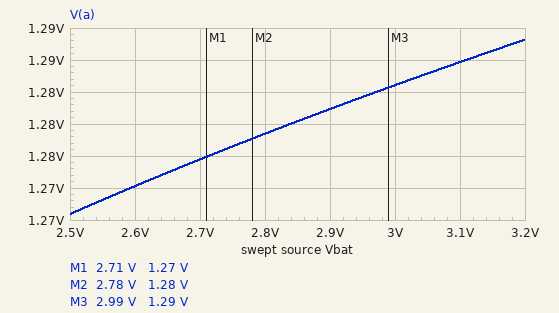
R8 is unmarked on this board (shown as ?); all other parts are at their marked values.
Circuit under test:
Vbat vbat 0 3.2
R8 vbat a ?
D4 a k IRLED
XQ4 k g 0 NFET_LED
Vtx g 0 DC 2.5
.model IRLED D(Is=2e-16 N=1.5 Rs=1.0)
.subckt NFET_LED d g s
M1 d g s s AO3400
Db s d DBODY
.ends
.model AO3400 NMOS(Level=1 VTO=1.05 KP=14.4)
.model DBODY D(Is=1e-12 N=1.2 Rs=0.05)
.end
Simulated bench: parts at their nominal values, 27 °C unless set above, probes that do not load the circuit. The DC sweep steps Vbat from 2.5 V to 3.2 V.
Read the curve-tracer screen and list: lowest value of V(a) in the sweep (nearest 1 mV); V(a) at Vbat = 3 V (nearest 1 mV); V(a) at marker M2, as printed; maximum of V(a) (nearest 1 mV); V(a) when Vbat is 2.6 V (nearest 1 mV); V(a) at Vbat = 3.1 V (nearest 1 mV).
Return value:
1.266 V
1.286 V
1.28 V
1.293 V
1.270 V
1.290 V
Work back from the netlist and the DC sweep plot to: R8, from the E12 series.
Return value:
68 Ω
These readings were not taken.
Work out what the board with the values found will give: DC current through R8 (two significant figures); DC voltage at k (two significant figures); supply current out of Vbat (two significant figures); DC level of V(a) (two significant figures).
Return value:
28 mA
1.3 mV
28 mA
1.3 V
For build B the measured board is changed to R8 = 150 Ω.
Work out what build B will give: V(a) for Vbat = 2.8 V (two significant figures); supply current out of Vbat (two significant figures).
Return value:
1.2 V
13 mA
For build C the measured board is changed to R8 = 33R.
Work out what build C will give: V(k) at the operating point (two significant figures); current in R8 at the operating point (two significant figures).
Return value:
2.7 mV
56 mA
